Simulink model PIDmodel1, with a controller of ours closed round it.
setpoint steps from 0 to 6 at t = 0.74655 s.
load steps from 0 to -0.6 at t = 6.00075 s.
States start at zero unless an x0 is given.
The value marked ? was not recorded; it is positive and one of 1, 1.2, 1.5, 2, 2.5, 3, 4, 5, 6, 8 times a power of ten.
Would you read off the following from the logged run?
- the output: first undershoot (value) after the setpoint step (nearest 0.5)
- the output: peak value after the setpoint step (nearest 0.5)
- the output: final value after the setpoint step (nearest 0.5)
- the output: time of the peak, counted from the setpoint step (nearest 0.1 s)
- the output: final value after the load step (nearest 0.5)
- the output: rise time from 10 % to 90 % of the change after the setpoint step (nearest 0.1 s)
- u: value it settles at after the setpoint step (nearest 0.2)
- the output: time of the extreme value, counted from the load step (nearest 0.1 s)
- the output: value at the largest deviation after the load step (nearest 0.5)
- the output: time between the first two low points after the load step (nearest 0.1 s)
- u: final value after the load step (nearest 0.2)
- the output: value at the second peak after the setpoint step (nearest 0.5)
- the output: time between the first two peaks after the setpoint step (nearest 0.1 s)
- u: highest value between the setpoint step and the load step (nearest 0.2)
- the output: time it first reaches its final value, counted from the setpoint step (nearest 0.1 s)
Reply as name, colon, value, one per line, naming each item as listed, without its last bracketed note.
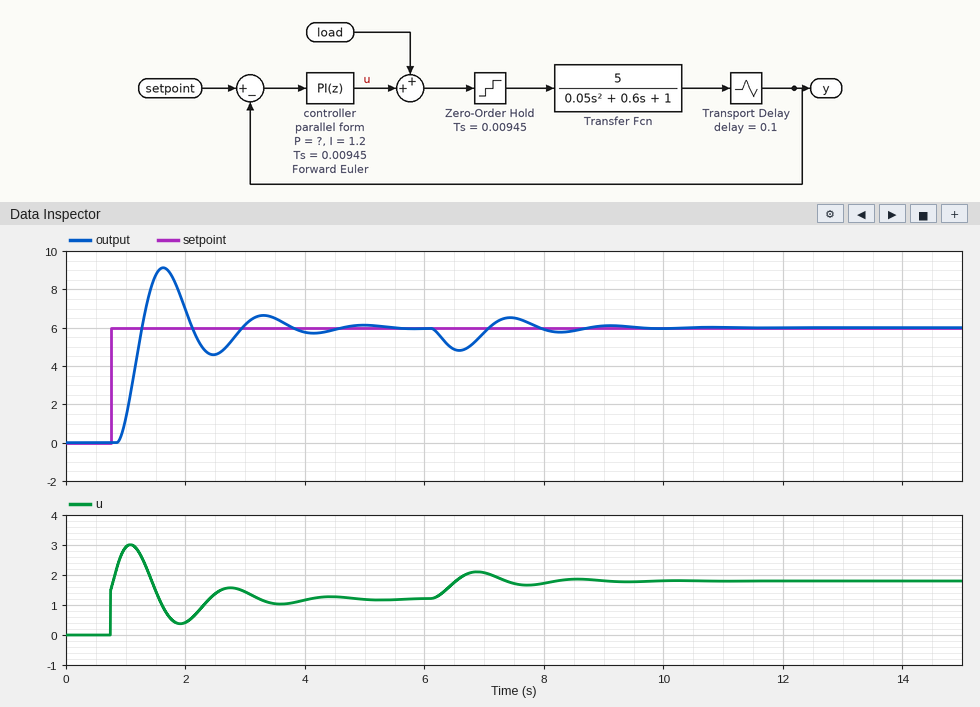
the output: first undershoot (value) after the setpoint step: 4.5
the output: peak value after the setpoint step: 9.0
the output: final value after the setpoint step: 6.0
the output: time of the peak, counted from the setpoint step: 0.9 s
the output: final value after the load step: 6.0
the output: rise time from 10 % to 90 % of the change after the setpoint step: 0.3 s
u: value it settles at after the setpoint step: 1.2
the output: time of the extreme value, counted from the load step: 0.6 s
the output: value at the largest deviation after the load step: 5.0
the output: time between the first two low points after the load step: 1.7 s
u: final value after the load step: 1.8
the output: value at the second peak after the setpoint step: 6.5
the output: time between the first two peaks after the setpoint step: 1.7 s
u: highest value between the setpoint step and the load step: 3.0
the output: time it first reaches its final value, counted from the setpoint step: 0.5 s
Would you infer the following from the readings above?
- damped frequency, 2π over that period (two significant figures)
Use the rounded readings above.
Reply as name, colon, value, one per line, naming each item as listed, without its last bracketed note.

damped frequency, 2π over that period: 3.7 rad/s
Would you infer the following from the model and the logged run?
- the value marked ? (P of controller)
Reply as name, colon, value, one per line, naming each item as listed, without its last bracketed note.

the value marked ?: 0.25
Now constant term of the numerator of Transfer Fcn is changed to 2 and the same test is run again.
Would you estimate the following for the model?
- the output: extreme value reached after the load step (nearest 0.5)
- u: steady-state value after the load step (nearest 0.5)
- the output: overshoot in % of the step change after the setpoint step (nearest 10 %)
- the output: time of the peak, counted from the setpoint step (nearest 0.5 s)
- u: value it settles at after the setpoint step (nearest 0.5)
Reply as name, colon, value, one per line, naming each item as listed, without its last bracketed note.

the output: extreme value reached after the load step: 5.5
u: steady-state value after the load step: 3.5
the output: overshoot in % of the step change after the setpoint step: 20 %
the output: time of the peak, counted from the setpoint step: 1.5 s
u: value it settles at after the setpoint step: 3.0
